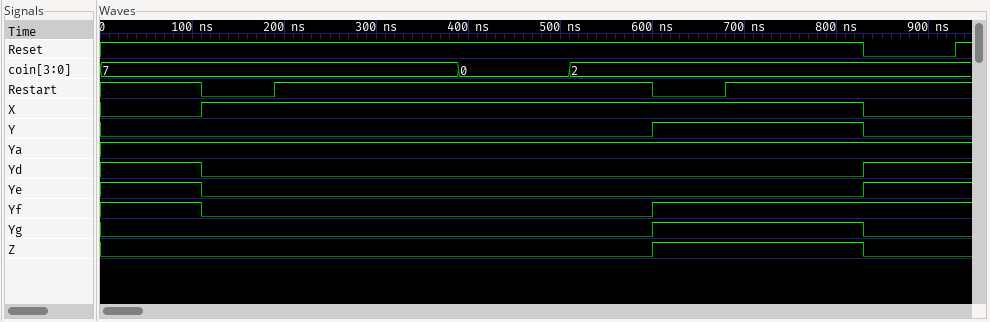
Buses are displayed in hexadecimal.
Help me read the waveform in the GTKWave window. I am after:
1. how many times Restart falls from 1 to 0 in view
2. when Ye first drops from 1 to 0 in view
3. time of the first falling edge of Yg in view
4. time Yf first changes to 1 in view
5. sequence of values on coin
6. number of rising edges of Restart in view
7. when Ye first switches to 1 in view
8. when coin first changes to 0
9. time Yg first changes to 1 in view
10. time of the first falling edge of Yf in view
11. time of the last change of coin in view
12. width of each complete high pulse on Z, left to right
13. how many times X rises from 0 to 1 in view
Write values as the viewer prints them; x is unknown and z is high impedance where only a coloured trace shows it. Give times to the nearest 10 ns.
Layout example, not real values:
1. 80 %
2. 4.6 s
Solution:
1. 2
2. 110 ns
3. 830 ns
4. 600 ns
5. 7, 0, 2
6. 2
7. 830 ns
8. 390 ns
9. 600 ns
10. 110 ns
11. 510 ns
12. 230 ns
13. 1
